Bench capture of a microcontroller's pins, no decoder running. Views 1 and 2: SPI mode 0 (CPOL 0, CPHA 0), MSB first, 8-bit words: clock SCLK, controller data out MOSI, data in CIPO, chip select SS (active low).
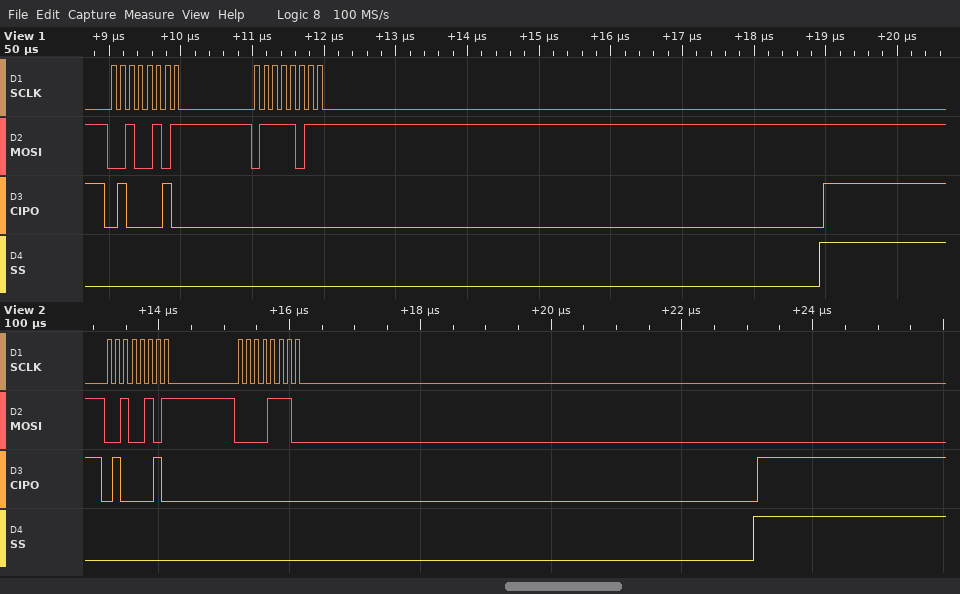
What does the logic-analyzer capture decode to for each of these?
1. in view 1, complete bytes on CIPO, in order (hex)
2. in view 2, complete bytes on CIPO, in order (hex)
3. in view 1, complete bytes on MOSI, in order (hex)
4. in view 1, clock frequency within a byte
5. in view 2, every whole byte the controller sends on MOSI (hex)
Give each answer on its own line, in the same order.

0x42 0x00
42 00
0x25 0x7B
8 MHz
25 0E
